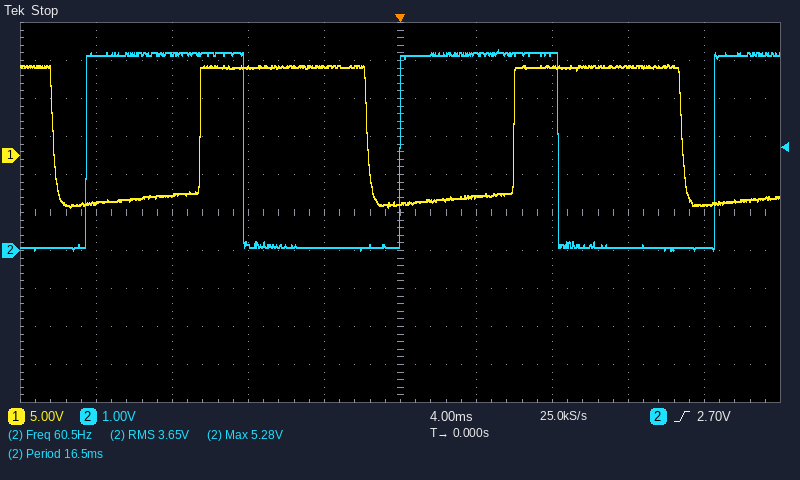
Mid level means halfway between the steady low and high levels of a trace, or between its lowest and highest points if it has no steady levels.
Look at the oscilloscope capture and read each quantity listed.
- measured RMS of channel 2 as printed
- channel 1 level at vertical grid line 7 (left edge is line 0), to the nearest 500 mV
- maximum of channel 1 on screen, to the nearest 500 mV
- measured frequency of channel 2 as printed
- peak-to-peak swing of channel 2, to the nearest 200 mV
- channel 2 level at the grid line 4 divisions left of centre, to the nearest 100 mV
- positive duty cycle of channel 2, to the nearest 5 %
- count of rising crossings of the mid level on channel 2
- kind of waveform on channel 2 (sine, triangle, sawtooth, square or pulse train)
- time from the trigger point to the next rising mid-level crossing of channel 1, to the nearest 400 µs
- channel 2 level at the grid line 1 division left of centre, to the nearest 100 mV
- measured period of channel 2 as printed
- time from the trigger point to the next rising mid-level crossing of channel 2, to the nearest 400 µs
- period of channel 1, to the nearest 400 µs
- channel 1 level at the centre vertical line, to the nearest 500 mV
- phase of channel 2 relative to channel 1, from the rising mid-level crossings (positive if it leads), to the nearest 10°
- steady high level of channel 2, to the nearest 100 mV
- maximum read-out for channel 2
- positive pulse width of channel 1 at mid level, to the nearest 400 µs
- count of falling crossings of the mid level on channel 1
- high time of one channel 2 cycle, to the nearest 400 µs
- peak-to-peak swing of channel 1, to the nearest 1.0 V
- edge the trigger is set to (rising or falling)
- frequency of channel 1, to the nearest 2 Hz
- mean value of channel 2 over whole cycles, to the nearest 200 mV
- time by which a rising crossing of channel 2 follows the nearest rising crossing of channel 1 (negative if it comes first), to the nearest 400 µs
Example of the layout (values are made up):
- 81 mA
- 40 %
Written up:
- 3.65 V
- 11.5 V
- 12.0 V
- 60.5 Hz
- 5.2 V
- 5.1 V
- 50 %
- 3
- square
- 6.0 ms
- 100 mV
- 16.5 ms
- 16.4 ms
- 16.4 ms
- -6.5 V
- +130°
- 5.2 V
- 5.28 V
- 8.8 ms
- 3
- 8.4 ms
- 19.0 V
- rising
- 60 Hz
- 2.6 V
- -6.0 ms
